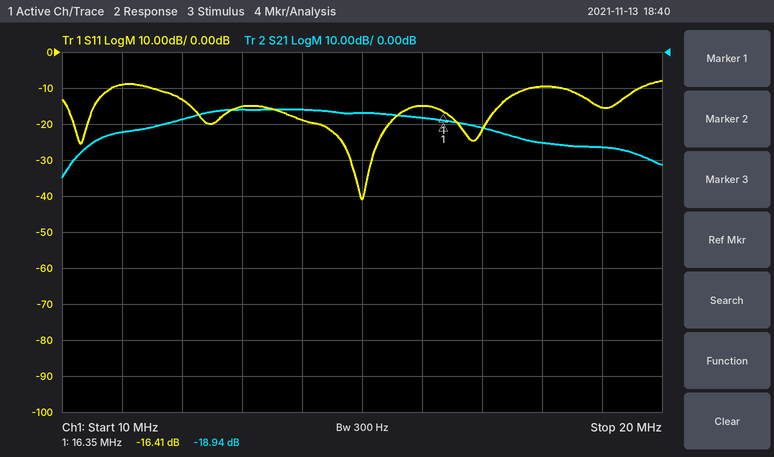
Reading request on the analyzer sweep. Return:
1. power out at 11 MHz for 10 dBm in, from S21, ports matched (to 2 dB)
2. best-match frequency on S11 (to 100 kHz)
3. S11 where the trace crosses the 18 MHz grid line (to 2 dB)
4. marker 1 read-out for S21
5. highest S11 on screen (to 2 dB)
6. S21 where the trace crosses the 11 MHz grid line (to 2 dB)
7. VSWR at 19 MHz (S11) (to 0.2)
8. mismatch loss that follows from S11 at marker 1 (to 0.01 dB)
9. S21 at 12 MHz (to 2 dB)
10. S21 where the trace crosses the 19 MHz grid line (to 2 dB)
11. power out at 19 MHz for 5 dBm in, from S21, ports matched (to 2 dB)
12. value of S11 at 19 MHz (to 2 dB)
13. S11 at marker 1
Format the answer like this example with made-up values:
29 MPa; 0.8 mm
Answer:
-12 dBm; 15.0 MHz; -10 dB; -18.94 dB; -8 dB; -22 dB; 1.4; 0.10 dB; -18 dB; -26 dB; -22 dBm; -16 dB; -16.41 dB
